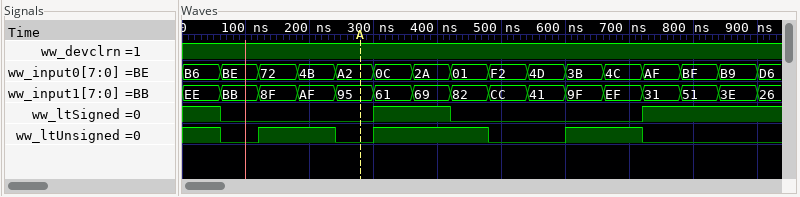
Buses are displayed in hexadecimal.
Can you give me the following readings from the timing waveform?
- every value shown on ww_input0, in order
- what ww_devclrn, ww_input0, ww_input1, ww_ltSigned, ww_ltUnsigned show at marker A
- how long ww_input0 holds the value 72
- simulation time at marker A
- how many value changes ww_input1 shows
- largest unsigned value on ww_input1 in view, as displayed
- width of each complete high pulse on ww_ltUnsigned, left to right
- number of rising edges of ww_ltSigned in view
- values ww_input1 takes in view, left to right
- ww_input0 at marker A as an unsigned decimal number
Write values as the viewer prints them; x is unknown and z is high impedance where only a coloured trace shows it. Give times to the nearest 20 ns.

B6, BE, 72, 4B, A2, 0C, 2A, 01, F2, 4D, 3B, 4C, AF, BF, B9, D6
ww_devclrn=1, ww_input0=A2, ww_input1=95, ww_ltSigned=0, ww_ltUnsigned=0
60 ns
280 ns
15
EF
120 ns, 180 ns, 120 ns
2
EE, BB, 8F, AF, 95, 61, 69, 82, CC, 41, 9F, EF, 31, 51, 3E, 26
162
